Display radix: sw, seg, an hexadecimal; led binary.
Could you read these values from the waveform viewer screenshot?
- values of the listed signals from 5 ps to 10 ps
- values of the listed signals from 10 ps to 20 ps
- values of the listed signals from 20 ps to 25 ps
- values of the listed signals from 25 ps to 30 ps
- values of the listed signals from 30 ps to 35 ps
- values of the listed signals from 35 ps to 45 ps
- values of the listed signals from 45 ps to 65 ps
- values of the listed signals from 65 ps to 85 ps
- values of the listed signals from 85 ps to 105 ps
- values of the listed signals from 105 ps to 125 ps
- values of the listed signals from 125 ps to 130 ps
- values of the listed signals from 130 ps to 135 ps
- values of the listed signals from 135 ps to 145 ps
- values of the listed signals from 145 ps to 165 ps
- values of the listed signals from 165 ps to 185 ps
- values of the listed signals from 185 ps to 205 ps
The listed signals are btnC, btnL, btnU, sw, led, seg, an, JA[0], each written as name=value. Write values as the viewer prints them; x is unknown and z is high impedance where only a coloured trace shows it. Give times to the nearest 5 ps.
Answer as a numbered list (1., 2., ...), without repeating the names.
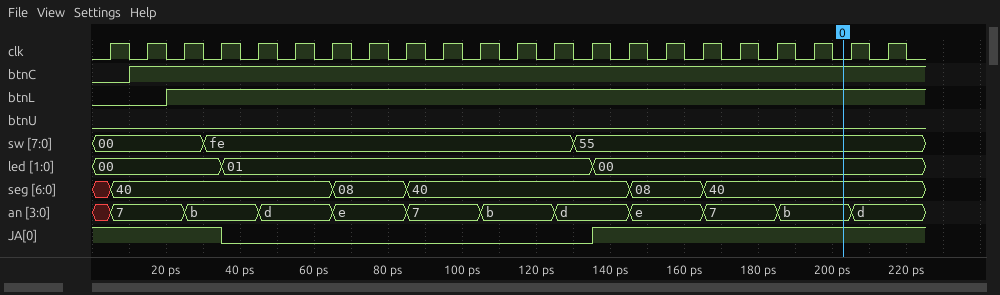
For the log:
1. btnC=0, btnL=0, btnU=0, sw=00, led=00, seg=40, an=7, JA[0]=1
2. btnC=1, btnL=0, btnU=0, sw=00, led=00, seg=40, an=7, JA[0]=1
3. btnC=1, btnL=1, btnU=0, sw=00, led=00, seg=40, an=7, JA[0]=1
4. btnC=1, btnL=1, btnU=0, sw=00, led=00, seg=40, an=b, JA[0]=1
5. btnC=1, btnL=1, btnU=0, sw=fe, led=00, seg=40, an=b, JA[0]=1
6. btnC=1, btnL=1, btnU=0, sw=fe, led=01, seg=40, an=b, JA[0]=0
7. btnC=1, btnL=1, btnU=0, sw=fe, led=01, seg=40, an=d, JA[0]=0
8. btnC=1, btnL=1, btnU=0, sw=fe, led=01, seg=08, an=e, JA[0]=0
9. btnC=1, btnL=1, btnU=0, sw=fe, led=01, seg=40, an=7, JA[0]=0
10. btnC=1, btnL=1, btnU=0, sw=fe, led=01, seg=40, an=b, JA[0]=0
11. btnC=1, btnL=1, btnU=0, sw=fe, led=01, seg=40, an=d, JA[0]=0
12. btnC=1, btnL=1, btnU=0, sw=55, led=01, seg=40, an=d, JA[0]=0
13. btnC=1, btnL=1, btnU=0, sw=55, led=00, seg=40, an=d, JA[0]=1
14. btnC=1, btnL=1, btnU=0, sw=55, led=00, seg=08, an=e, JA[0]=1
15. btnC=1, btnL=1, btnU=0, sw=55, led=00, seg=40, an=7, JA[0]=1
16. btnC=1, btnL=1, btnU=0, sw=55, led=00, seg=40, an=b, JA[0]=1
